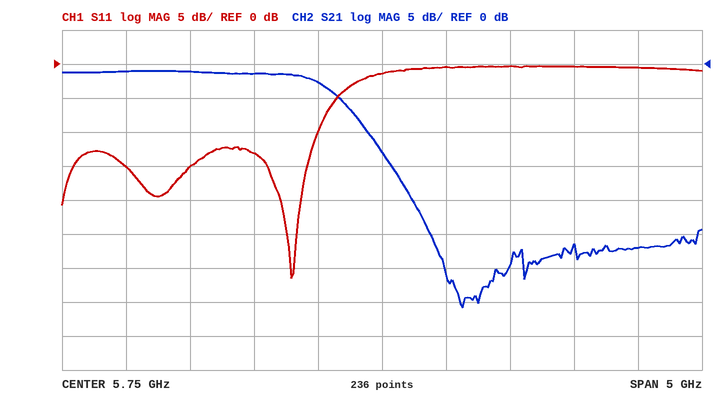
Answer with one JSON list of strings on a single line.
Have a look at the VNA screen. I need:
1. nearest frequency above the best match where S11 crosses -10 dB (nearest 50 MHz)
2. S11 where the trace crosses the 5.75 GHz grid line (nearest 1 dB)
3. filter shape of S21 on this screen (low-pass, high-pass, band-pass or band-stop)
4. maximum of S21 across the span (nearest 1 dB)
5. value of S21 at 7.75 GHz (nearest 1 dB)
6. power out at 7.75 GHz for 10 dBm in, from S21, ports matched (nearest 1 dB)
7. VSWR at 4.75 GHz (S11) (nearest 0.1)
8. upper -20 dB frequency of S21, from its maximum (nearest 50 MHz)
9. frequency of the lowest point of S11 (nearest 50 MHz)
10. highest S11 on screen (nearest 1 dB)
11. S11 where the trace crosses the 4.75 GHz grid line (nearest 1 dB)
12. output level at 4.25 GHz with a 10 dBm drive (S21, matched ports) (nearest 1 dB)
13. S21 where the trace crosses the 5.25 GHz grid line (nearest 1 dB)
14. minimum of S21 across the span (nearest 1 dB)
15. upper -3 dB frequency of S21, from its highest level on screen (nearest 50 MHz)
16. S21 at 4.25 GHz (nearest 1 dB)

["5.25 GHz", "-1 dB", "low-pass", "-1 dB", "-27 dB", "-17 dBm", "1.6", "6.00 GHz", "5.05 GHz", "0 dB", "-13 dB", "9 dBm", "-3 dB", "-36 dB", "5.35 GHz", "-1 dB"]
